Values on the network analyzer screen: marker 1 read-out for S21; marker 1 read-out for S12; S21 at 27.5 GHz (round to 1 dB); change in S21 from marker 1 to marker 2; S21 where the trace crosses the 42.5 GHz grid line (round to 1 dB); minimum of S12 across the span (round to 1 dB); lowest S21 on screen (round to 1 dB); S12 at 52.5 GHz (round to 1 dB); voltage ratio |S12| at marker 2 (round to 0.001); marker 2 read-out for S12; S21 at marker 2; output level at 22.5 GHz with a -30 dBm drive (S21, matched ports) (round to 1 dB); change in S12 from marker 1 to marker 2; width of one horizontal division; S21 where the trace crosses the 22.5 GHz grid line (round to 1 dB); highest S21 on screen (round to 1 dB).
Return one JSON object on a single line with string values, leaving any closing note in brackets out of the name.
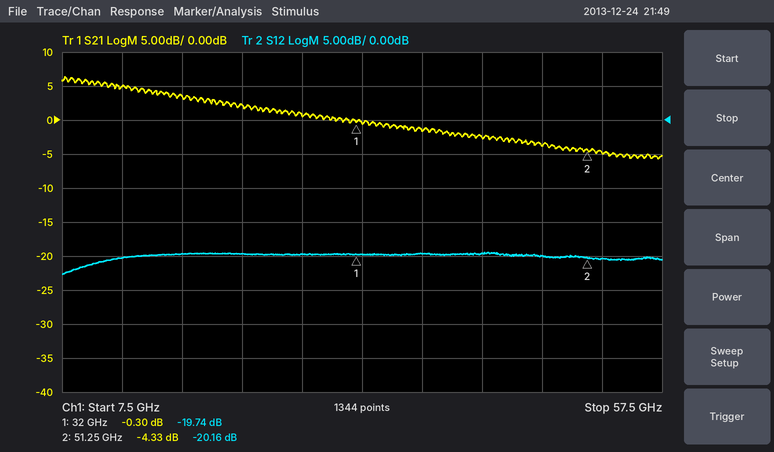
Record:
{"marker 1 read-out for S21": "-0.30 dB", "marker 1 read-out for S12": "-19.74 dB", "S21 at 27.5 GHz": "1 dB", "change in S21 from marker 1 to marker 2": "-4.03 dB", "S21 where the trace crosses the 42.5 GHz grid line": "-3 dB", "minimum of S12 across the span": "-23 dB", "lowest S21 on screen": "-6 dB", "S12 at 52.5 GHz": "-20 dB", "voltage ratio |S12| at marker 2": "0.098", "marker 2 read-out for S12": "-20.16 dB", "S21 at marker 2": "-4.33 dB", "output level at 22.5 GHz with a -30 dBm drive (S21, matched ports)": "-28 dBm", "change in S12 from marker 1 to marker 2": "-0.42 dB", "width of one horizontal division": "5 GHz", "S21 where the trace crosses the 22.5 GHz grid line": "2 dB", "highest S21 on screen": "6 dB"}
